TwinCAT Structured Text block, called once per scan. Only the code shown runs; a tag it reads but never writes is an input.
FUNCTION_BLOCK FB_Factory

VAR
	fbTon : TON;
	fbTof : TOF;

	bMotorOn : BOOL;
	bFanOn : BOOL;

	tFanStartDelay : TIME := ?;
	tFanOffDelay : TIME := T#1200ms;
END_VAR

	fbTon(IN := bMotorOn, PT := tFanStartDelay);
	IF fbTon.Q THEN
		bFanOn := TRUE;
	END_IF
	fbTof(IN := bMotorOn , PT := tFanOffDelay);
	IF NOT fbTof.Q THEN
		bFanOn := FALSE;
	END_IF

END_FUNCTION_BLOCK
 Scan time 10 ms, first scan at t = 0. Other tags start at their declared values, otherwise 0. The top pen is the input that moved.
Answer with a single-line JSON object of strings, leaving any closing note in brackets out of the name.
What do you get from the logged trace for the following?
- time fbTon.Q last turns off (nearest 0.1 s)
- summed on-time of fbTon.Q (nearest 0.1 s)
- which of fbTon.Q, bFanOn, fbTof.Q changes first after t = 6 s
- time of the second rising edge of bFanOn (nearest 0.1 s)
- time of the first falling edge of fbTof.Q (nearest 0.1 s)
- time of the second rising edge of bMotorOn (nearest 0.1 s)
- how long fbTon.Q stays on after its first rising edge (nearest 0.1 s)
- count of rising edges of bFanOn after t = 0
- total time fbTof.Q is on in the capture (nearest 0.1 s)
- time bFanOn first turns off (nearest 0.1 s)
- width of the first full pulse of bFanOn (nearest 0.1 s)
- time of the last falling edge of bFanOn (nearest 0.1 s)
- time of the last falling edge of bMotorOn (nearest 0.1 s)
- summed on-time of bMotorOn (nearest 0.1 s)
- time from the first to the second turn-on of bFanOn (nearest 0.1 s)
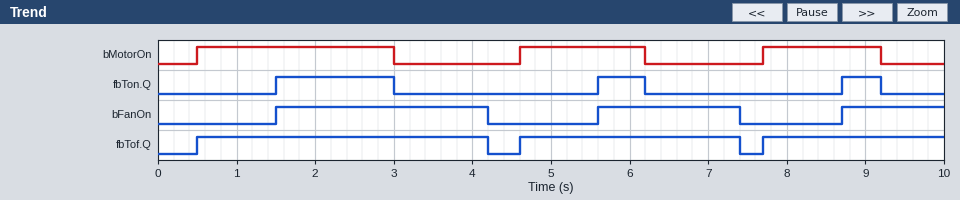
{"time fbTon.Q last turns off": "9.2 s", "summed on-time of fbTon.Q": "2.6 s", "which of fbTon.Q, bFanOn, fbTof.Q changes first after t = 6 s": "fbTon.Q", "time of the second rising edge of bFanOn": "5.6 s", "time of the first falling edge of fbTof.Q": "4.2 s", "time of the second rising edge of bMotorOn": "4.6 s", "how long fbTon.Q stays on after its first rising edge": "1.5 s", "count of rising edges of bFanOn after t = 0": "3", "total time fbTof.Q is on in the capture": "8.8 s", "time bFanOn first turns off": "4.2 s", "width of the first full pulse of bFanOn": "2.7 s", "time of the last falling edge of bFanOn": "7.4 s", "time of the last falling edge of bMotorOn": "9.2 s", "summed on-time of bMotorOn": "5.6 s", "time from the first to the second turn-on of bFanOn": "4.1 s"}
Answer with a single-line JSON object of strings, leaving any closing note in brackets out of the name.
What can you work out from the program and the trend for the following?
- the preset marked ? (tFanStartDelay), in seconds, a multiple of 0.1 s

{"the preset marked ? (tFanStartDelay), in seconds, a multiple of 0.1 s": "1.0 s"}
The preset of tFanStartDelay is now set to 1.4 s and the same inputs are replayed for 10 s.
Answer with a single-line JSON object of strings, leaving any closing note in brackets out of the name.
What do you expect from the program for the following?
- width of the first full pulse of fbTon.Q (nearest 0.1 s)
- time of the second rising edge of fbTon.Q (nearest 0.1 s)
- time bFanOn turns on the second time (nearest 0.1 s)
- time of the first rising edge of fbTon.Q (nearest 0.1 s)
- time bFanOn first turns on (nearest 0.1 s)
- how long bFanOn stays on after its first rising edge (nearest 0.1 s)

{"width of the first full pulse of fbTon.Q": "1.1 s", "time of the second rising edge of fbTon.Q": "6.0 s", "time bFanOn turns on the second time": "6.0 s", "time of the first rising edge of fbTon.Q": "1.9 s", "time bFanOn first turns on": "1.9 s", "how long bFanOn stays on after its first rising edge": "2.3 s"}
